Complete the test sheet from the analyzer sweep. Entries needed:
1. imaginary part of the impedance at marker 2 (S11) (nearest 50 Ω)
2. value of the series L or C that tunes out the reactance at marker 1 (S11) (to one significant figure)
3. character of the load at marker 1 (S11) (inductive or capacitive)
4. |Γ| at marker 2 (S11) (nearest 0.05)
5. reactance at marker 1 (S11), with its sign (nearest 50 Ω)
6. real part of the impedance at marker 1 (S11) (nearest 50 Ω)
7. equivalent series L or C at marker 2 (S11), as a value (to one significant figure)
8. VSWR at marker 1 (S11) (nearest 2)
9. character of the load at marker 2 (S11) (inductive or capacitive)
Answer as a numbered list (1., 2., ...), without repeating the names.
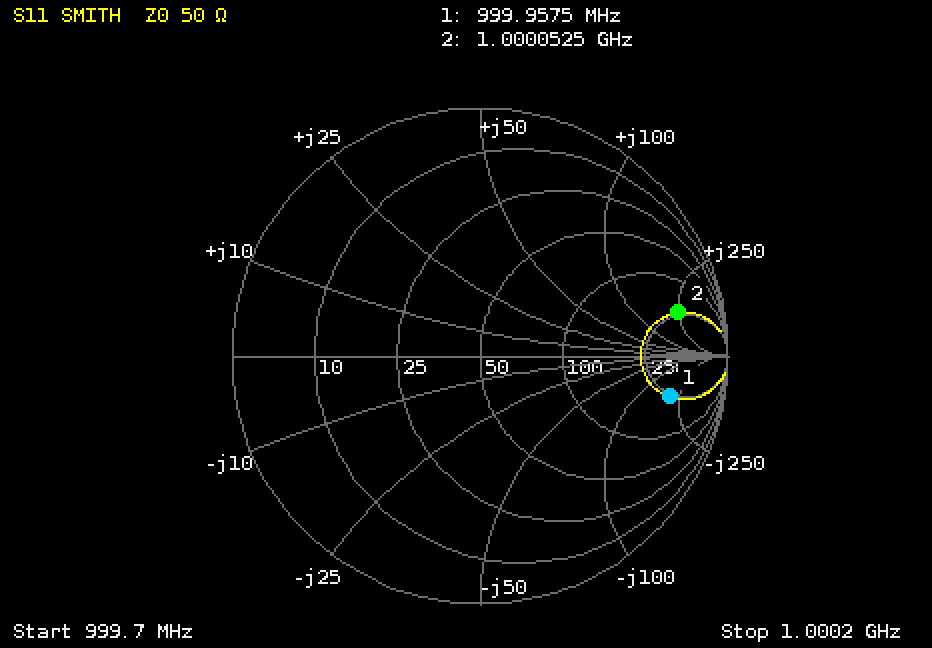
1. +250 Ω
2. 30 nH
3. capacitive
4. 0.80
5. -200 Ω
6. 250 Ω
7. 40 nH
8. 8
9. inductive
